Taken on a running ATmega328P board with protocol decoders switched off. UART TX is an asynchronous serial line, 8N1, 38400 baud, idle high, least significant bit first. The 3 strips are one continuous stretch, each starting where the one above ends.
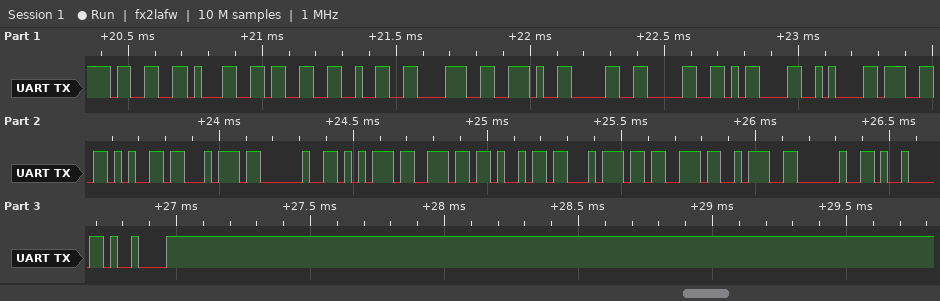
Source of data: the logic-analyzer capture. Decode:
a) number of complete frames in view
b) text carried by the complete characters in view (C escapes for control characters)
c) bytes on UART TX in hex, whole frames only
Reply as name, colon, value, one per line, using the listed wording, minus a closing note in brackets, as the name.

number of complete frames in view: 23
text carried by the complete characters in view: "31328.00\r\nget units: \t\t"
bytes on UART TX in hex, whole frames only: 33 31 33 32 38 2E 30 30 0D 0A 67 65 74 20 75 6E 69 74 73 3A 20 09 09
